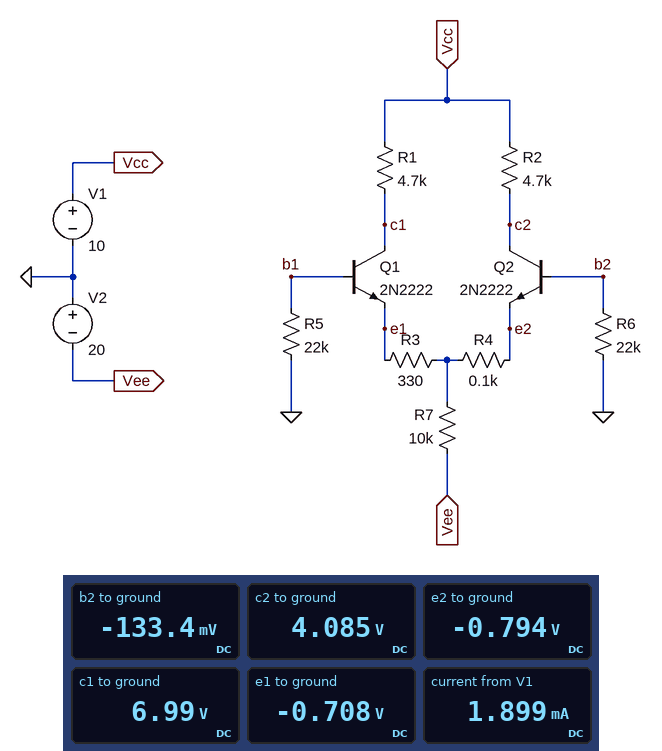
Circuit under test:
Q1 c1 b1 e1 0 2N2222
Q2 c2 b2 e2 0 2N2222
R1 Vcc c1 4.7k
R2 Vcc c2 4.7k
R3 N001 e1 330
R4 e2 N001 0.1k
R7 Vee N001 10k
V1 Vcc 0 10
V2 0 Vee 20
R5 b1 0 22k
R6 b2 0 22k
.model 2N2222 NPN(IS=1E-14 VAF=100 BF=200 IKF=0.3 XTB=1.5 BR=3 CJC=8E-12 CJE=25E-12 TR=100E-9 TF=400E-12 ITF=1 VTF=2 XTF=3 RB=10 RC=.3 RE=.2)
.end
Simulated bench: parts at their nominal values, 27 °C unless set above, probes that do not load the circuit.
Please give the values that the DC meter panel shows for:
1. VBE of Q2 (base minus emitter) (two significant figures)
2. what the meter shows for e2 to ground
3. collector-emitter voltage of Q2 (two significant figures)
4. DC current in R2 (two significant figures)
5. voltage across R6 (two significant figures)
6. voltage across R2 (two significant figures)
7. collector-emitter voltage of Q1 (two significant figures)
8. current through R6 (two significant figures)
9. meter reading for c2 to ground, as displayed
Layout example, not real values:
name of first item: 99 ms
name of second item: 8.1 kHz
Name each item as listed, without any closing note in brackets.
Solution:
VBE of Q2 (base minus emitter): 660 mV
what the meter shows for e2 to ground: -0.794 V
collector-emitter voltage of Q2: 4.9 V
DC current in R2: 1.3 mA
voltage across R6: 130 mV
voltage across R2: 5.9 V
collector-emitter voltage of Q1: 7.7 V
current through R6: 6.1 µA
meter reading for c2 to ground, as displayed: 4.085 V
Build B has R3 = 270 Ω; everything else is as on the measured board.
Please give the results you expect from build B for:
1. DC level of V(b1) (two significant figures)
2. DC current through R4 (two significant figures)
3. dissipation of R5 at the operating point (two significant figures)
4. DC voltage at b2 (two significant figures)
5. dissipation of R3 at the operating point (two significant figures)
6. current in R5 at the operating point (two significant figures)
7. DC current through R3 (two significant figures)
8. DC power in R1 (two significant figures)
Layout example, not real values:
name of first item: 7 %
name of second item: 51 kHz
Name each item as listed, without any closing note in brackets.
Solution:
DC level of V(b1): -72 mV
DC current through R4: 1.2 mA
dissipation of R5 at the operating point: 240 nW
DC voltage at b2: -130 mV
dissipation of R3 at the operating point: 130 µW
current in R5 at the operating point: 3.3 µA
DC current through R3: 700 µA
DC power in R1: 2.3 mW
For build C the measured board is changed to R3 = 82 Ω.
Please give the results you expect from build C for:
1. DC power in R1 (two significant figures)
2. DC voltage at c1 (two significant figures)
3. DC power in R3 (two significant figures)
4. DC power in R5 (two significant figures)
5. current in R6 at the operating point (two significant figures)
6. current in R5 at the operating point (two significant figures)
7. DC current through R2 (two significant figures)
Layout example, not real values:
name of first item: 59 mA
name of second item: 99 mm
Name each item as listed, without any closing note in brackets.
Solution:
DC power in R1: 4.6 mW
DC voltage at c1: 5.3 V
DC power in R3: 81 µW
DC power in R5: 490 nW
current in R6 at the operating point: 4.3 µA
current in R5 at the operating point: 4.7 µA
DC current through R2: 920 µA
